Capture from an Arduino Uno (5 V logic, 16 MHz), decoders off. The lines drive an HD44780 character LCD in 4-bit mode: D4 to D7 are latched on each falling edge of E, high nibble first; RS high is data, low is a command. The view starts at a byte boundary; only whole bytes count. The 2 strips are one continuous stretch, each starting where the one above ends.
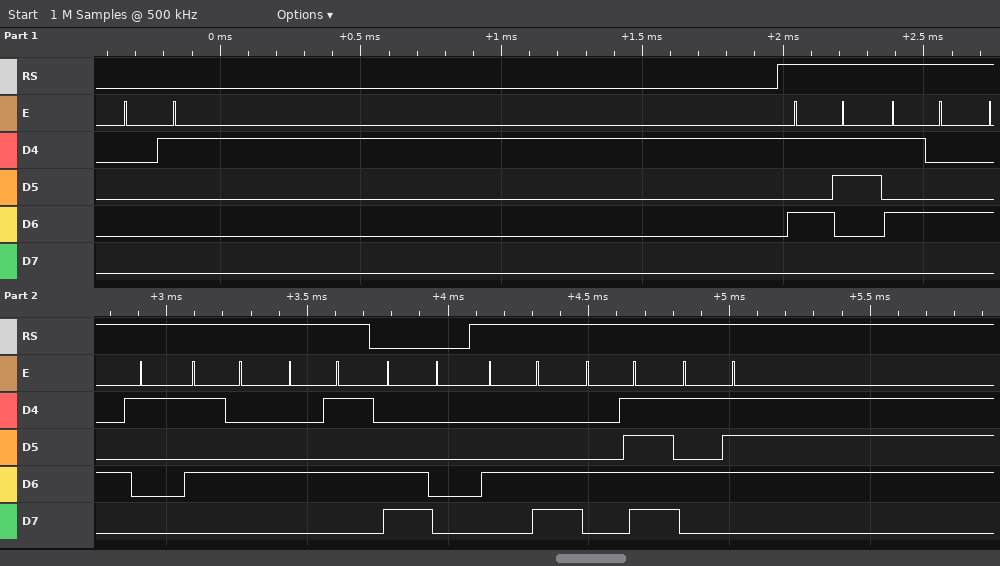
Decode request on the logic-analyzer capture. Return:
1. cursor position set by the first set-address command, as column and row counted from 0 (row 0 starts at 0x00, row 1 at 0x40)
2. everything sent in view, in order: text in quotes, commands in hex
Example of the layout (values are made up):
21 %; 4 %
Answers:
column 0, row 1; 0x01 "STATE" 0xC0 "LOW"
